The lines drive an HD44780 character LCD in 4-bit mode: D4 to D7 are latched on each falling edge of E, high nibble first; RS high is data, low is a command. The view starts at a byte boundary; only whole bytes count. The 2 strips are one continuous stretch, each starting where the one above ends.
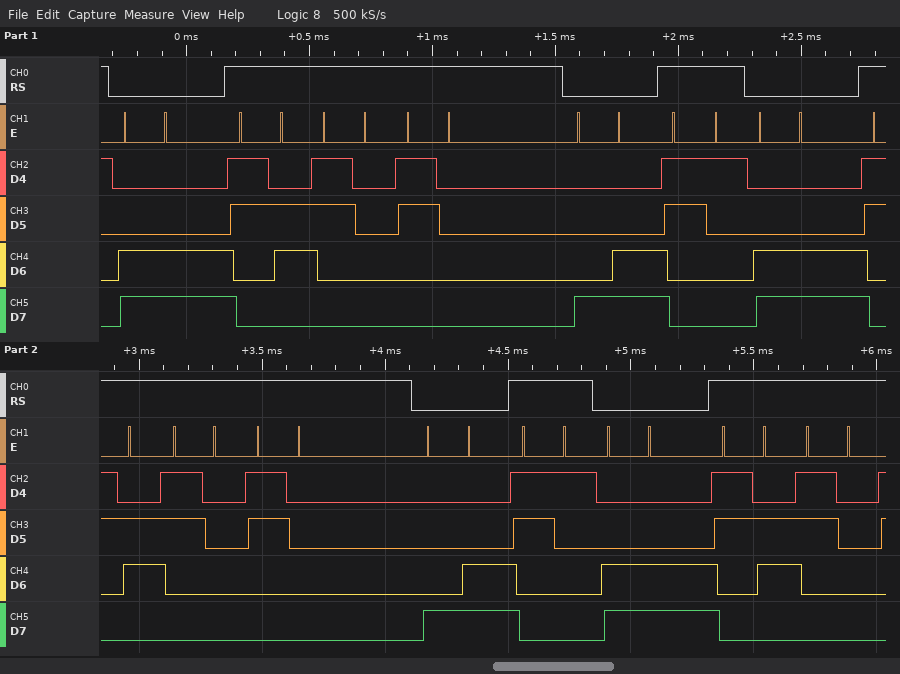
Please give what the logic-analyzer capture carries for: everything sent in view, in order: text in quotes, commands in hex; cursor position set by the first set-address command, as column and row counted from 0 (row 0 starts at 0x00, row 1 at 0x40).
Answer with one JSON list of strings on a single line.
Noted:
["0xCC \"600\" 0x8C \"1\" 0xCC \"600\" 0x8C \"1\" 0xCC \"60\"", "column 12, row 1"]
